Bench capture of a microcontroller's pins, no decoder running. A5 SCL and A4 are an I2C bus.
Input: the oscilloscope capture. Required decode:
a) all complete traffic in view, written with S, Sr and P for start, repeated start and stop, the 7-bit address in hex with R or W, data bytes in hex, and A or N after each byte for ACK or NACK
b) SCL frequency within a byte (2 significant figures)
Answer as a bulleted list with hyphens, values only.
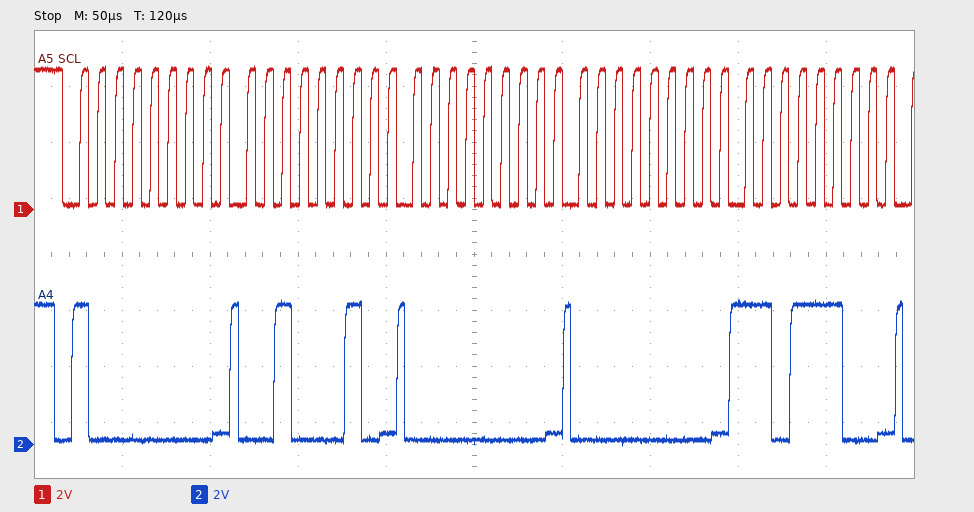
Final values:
- S 40W A 22 A 00 A 00 A DC A
- 100 kHz
